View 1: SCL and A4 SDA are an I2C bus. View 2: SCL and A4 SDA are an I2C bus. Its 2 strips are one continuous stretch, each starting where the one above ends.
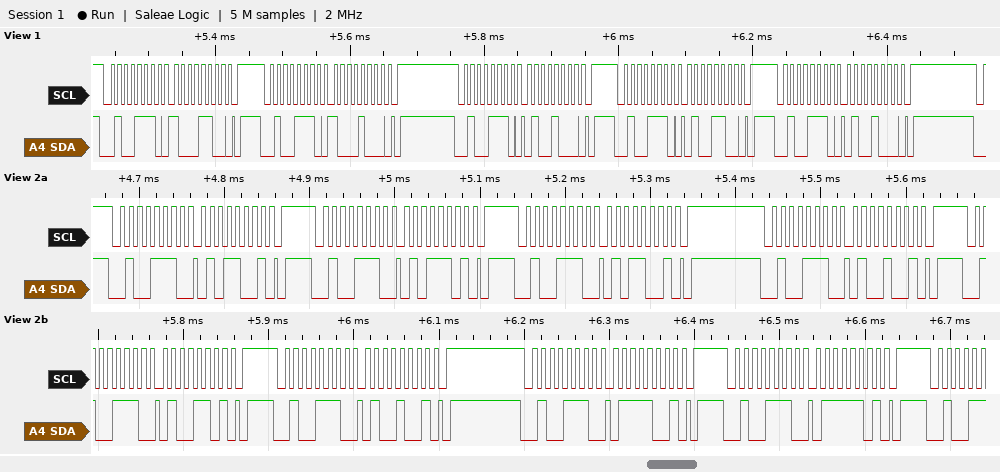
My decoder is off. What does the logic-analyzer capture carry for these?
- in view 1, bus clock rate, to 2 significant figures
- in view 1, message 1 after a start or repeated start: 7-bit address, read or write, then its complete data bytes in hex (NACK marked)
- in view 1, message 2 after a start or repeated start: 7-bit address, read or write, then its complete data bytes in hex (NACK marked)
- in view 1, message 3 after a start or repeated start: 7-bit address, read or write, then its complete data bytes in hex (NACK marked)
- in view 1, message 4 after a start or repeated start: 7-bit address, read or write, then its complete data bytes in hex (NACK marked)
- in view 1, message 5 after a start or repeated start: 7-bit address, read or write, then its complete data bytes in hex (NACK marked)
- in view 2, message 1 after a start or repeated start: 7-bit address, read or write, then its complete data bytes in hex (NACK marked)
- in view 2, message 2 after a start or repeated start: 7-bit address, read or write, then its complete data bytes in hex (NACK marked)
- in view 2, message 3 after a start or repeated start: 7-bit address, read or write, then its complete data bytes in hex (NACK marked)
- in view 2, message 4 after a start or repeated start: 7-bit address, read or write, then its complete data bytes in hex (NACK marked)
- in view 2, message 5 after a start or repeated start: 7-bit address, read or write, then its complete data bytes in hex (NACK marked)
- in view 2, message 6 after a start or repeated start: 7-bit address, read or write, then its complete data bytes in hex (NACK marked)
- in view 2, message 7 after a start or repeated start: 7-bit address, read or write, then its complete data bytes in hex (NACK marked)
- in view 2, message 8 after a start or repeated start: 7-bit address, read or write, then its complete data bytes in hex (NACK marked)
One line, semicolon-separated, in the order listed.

100 kHz; 0x27 write: 8C; 0x27 write: 88; 0x27 write: 48; 0x27 write: 4C; 0x27 write: 48; 0x27 write: 59; 0x27 write: 5D; 0x27 write: 59; 0x27 write: 49; 0x27 write: 4D; 0x27 write: 49; 0x27 write: 79; 0x27 write: 7D
